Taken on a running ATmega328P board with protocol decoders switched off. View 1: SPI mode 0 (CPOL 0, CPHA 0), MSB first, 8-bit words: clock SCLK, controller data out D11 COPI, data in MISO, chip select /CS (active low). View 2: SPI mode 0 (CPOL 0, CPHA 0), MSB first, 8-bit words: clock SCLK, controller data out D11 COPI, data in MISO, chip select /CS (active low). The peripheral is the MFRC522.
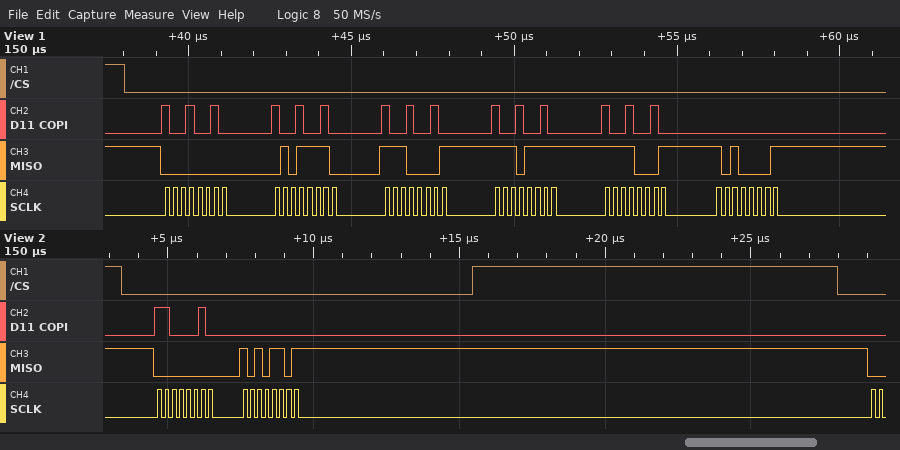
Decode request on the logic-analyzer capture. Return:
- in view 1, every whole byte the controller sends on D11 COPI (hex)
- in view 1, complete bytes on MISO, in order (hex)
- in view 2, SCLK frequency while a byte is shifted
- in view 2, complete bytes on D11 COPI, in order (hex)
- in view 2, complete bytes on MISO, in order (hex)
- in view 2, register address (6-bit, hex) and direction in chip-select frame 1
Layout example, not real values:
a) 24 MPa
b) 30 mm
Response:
a) 92 92 92 92 92 00
b) 00 5E E1 EF F1 A1
c) 4 MHz
d) C2 00
e) 00 AD
f) 0x21 read
